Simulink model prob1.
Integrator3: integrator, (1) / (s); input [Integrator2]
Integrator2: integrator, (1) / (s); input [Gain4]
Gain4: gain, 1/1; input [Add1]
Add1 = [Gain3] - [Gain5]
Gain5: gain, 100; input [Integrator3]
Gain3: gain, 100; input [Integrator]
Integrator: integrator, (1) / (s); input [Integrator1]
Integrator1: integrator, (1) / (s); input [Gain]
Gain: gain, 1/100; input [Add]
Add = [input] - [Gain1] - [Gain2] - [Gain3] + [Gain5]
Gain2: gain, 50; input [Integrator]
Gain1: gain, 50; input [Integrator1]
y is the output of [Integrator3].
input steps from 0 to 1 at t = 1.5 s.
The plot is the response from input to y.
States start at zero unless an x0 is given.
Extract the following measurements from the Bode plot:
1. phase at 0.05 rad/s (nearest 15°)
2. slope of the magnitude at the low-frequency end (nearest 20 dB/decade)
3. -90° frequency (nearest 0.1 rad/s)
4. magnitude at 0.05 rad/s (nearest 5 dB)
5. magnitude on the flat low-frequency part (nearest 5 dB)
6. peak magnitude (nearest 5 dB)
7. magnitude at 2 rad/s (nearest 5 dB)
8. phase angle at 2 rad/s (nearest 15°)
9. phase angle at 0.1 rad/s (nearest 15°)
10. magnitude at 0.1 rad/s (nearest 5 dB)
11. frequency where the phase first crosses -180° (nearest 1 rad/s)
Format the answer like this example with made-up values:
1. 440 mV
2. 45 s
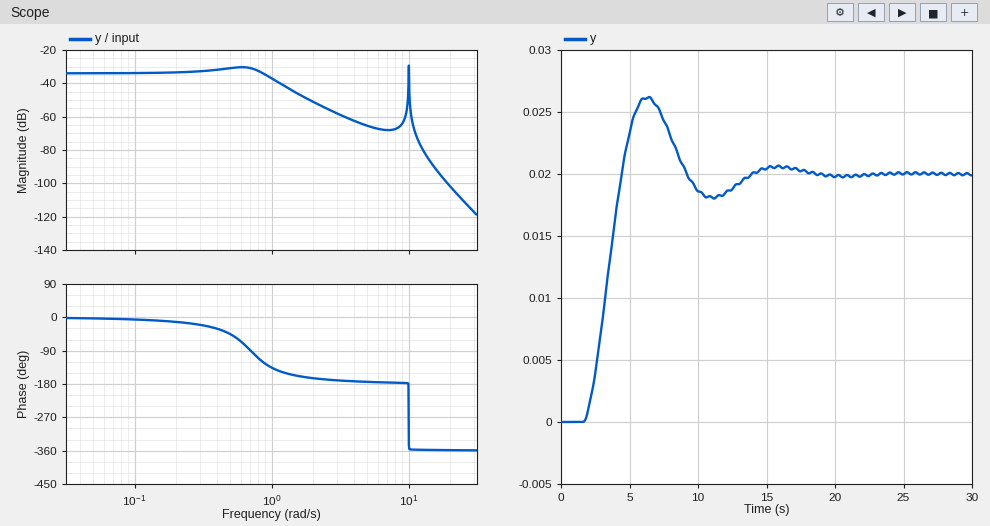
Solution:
1. 0°
2. 0 dB/decade
3. 0.7 rad/s
4. -35 dB
5. -35 dB
6. -30 dB
7. -50 dB
8. -165°
9. 0°
10. -35 dB
11. 10 rad/s
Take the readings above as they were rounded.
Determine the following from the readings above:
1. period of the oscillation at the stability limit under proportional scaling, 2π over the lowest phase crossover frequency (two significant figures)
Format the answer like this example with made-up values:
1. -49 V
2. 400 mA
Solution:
1. 0.63 s
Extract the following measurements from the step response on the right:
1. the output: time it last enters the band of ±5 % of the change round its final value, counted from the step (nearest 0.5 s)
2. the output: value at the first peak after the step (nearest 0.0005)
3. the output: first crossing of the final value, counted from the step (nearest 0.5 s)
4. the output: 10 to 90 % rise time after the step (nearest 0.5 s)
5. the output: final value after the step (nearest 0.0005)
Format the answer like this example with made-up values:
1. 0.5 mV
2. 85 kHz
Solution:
1. 11.0 s
2. 0.0260
3. 3.0 s
4. 2.0 s
5. 0.0200
